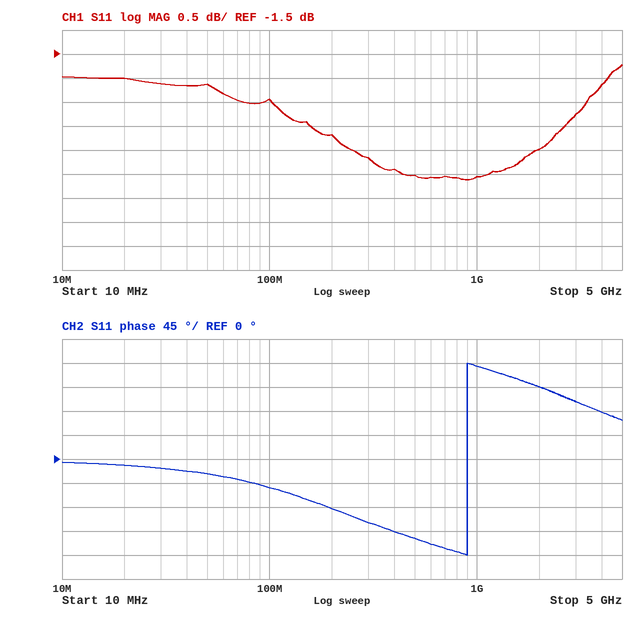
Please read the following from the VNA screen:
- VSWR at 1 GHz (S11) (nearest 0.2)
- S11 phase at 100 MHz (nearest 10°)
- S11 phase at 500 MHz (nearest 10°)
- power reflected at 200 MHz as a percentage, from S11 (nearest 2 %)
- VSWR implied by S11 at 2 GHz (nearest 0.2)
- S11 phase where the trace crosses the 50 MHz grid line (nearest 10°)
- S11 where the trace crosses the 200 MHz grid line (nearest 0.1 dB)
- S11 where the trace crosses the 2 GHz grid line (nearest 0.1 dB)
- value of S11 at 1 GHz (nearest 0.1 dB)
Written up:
4.4
-50°
-150°
48 %
5.0
-30°
-3.2 dB
-3.5 dB
-4.1 dB
